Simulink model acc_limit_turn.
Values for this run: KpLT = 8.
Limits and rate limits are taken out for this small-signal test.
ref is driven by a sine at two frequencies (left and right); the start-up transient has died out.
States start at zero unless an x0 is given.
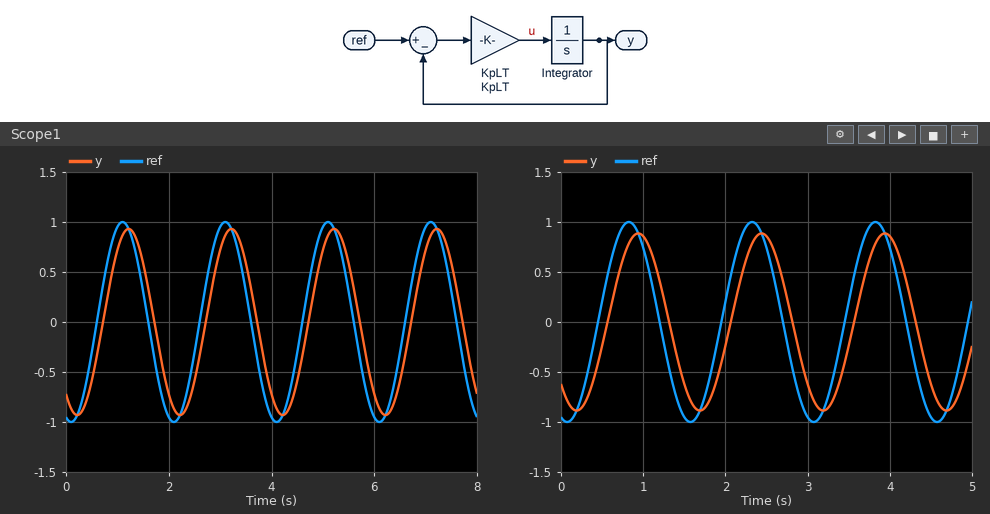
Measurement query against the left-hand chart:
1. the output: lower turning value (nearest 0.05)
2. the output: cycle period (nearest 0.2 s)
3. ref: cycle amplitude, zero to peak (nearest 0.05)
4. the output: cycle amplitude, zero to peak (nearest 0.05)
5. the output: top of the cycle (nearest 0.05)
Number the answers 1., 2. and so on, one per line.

1. -0.95
2. 2.0 s
3. 1.00
4. 0.95
5. 0.95
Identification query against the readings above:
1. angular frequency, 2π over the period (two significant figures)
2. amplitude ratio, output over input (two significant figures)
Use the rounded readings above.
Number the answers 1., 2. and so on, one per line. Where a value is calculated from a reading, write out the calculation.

1. 2π / 2 = 3.1 rad/s
2. 0.95 / 1 = 0.95
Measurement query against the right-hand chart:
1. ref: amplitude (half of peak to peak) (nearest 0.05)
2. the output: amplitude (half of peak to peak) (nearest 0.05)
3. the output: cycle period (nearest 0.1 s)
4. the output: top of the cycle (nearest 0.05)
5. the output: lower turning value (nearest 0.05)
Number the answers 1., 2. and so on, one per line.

1. 1.00
2. 0.90
3. 1.5 s
4. 0.90
5. -0.90
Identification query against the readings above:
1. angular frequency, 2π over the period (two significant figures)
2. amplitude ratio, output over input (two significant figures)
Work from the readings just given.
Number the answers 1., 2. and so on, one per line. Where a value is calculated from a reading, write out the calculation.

1. 2π / 1.5 = 4.2 rad/s
2. 0.9 / 1 = 0.90
